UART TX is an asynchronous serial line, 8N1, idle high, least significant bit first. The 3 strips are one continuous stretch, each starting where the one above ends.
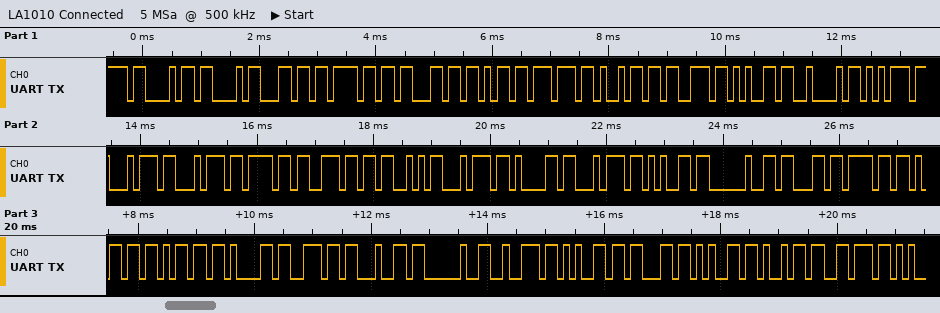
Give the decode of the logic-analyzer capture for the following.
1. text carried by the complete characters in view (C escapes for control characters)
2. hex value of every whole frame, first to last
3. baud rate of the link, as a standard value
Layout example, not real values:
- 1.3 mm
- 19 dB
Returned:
- "CClockwiseButtonState command receiv"
- 0x43 0x43 0x6C 0x6F 0x63 0x6B 0x77 0x69 0x73 0x65 0x42 0x75 0x74 0x74 0x6F 0x6E 0x53 0x74 0x61 0x74 0x65 0x20 0x63 0x6F 0x6D 0x6D 0x61 0x6E 0x64 0x20 0x72 0x65 0x63 0x65 0x69 0x76
- 9600 baud
